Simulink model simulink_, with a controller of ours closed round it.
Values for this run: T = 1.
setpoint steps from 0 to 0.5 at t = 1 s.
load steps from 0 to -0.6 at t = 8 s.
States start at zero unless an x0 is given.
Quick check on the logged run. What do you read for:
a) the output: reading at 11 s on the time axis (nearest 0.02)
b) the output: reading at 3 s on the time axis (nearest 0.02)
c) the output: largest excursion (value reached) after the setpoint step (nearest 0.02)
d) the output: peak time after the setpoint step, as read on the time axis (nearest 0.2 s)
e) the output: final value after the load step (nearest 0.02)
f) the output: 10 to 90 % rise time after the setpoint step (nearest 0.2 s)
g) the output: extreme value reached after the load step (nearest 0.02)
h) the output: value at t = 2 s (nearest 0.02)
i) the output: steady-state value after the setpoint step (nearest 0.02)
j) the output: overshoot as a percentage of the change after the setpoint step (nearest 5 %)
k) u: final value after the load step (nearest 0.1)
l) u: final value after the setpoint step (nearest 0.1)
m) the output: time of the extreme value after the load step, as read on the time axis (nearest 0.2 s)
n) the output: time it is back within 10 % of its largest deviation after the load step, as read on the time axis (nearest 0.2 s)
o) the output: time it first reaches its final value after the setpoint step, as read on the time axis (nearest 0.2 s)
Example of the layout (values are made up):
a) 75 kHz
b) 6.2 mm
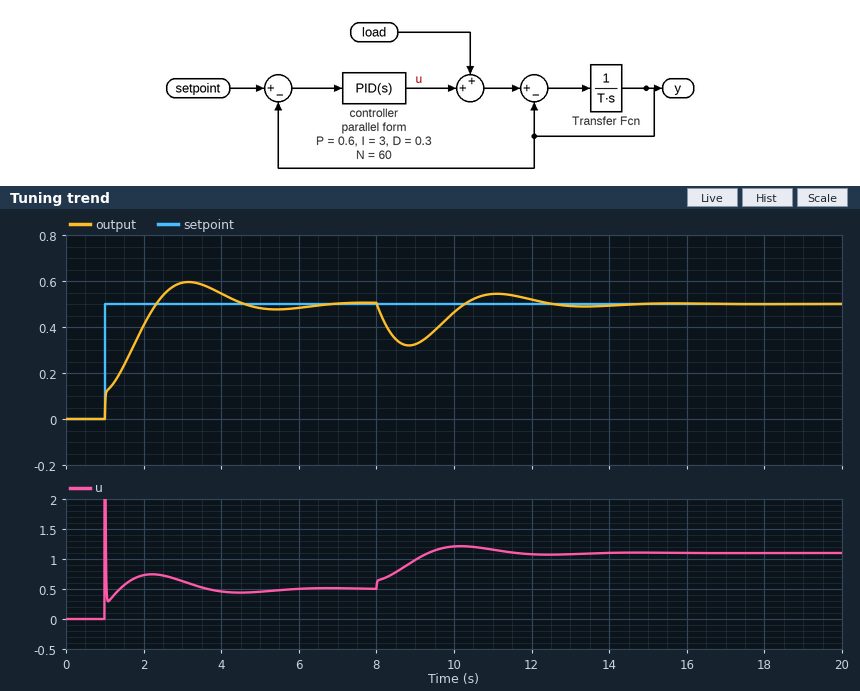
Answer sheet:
a) 0.54
b) 0.60
c) 0.60
d) 3.2 s
e) 0.50
f) 1.2 s
g) 0.32
h) 0.40
i) 0.50
j) 20 %
k) 1.1
l) 0.5
m) 8.8 s
n) 12.0 s
o) 2.4 s
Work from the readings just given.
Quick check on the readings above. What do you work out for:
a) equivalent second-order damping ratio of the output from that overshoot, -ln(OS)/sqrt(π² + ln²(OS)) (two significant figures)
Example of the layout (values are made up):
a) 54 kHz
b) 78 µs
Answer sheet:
a) 0.46
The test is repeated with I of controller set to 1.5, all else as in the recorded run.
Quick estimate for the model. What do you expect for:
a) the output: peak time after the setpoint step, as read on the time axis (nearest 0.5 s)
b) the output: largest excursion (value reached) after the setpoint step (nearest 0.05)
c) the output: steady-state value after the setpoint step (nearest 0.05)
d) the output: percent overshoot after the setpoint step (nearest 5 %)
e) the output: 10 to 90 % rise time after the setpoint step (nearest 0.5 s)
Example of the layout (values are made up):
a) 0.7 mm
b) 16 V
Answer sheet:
a) 4.5 s
b) 0.55
c) 0.50
d) 10 %
e) 2.0 s
